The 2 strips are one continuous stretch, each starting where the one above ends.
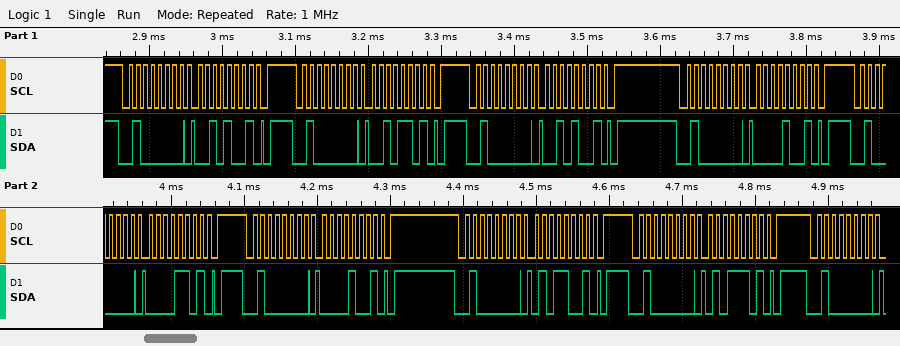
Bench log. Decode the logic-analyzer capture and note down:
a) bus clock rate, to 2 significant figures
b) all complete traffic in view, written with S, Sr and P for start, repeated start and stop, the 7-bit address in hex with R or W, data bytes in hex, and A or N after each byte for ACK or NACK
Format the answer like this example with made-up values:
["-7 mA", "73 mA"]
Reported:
["100 kHz", "S 20W A 29 A P S 20W A 2D A P S 20W A 29 A P S 20W A 09 A P S 20W A 0D A P S 20W A 09 A P S 20W A 59 A P S 20W A 5D A P S 20W A"]
